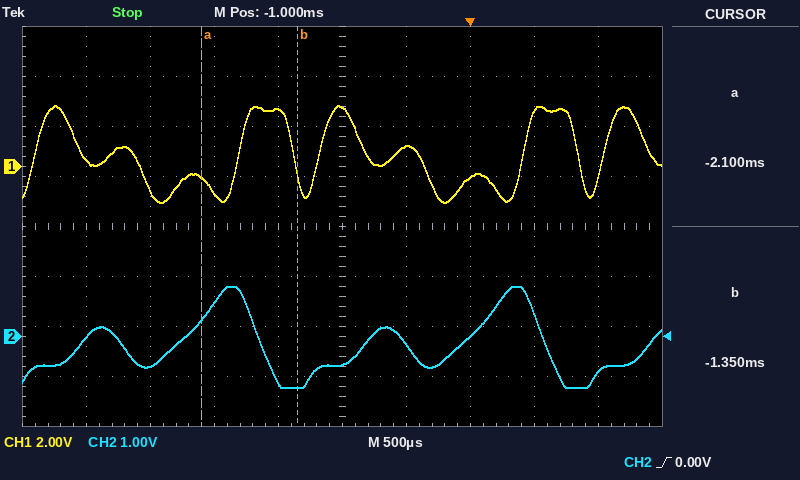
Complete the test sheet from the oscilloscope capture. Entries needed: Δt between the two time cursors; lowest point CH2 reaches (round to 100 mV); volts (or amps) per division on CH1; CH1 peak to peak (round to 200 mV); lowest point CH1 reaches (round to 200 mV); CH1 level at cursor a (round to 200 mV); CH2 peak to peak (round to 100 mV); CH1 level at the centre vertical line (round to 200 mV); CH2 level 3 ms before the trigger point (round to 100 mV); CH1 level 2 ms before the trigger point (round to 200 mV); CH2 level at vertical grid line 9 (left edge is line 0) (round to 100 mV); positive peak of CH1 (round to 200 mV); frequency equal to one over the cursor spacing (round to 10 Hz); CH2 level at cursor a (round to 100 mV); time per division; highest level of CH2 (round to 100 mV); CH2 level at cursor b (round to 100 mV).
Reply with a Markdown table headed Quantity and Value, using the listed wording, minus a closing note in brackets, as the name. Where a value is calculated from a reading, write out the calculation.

| Quantity | Value |
|---|---|
| Δt between the two time cursors | -1.35 ms − (-2.1 ms) = 750 µs |
| lowest point CH2 reaches | -1.0 V |
| volts (or amps) per division on CH1 | 2 V |
| CH1 peak to peak | 2.4 V − (-1.4 V) = 3.8 V |
| lowest point CH1 reaches | -1.4 V |
| CH1 level at cursor a | -400 mV |
| CH2 peak to peak | 1.0 V − (-1.0 V) = 2.0 V |
| CH1 level at the centre vertical line | 2.4 V |
| CH2 level 3 ms before the trigger point | 0.0 V |
| CH1 level 2 ms before the trigger point | -1.0 V |
| CH2 level at vertical grid line 9 (left edge is line 0) | -700 mV |
| positive peak of CH1 | 2.4 V |
| frequency equal to one over the cursor spacing | 1 / 750 µs ≈ 1.33 kHz |
| CH2 level at cursor a | 300 mV |
| time per division | 500 µs |
| highest level of CH2 | 1.0 V |
| CH2 level at cursor b | -1.0 V |
